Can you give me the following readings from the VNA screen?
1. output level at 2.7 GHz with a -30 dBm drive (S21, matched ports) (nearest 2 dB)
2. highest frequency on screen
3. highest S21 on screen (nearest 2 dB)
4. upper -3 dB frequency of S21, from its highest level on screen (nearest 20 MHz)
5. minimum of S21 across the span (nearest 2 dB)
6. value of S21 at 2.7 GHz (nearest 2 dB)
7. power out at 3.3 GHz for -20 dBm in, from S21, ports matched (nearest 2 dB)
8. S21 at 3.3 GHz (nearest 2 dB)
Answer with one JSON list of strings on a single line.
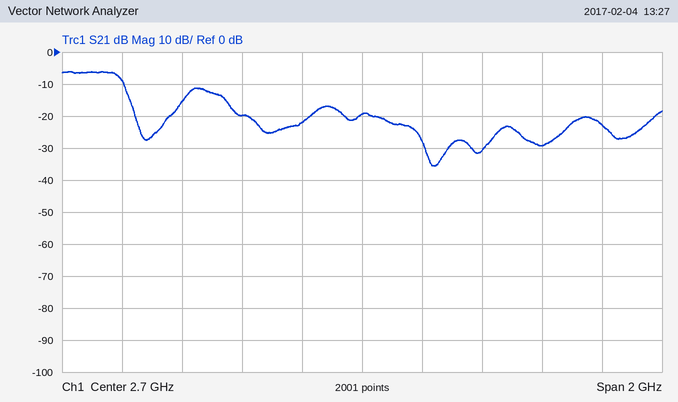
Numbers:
["-50 dBm", "3.7 GHz", "-6 dB", "1.90 GHz", "-36 dB", "-20 dB", "-50 dBm", "-30 dB"]
